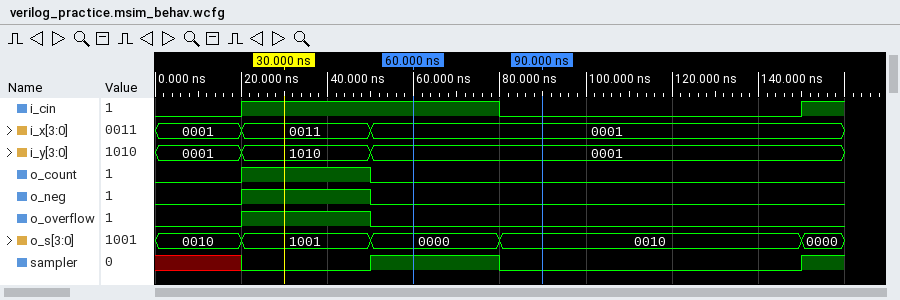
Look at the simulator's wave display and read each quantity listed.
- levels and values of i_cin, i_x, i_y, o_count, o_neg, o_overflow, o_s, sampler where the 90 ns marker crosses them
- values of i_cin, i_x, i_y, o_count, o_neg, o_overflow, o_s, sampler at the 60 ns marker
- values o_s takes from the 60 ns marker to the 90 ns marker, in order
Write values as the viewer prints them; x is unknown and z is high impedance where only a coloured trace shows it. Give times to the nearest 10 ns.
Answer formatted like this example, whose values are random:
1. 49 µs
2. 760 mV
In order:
1. i_cin=0, i_x=0001, i_y=0001, o_count=0, o_neg=0, o_overflow=0, o_s=0010, sampler=0
2. i_cin=1, i_x=0001, i_y=0001, o_count=0, o_neg=0, o_overflow=0, o_s=0000, sampler=1
3. 0000, 0010
